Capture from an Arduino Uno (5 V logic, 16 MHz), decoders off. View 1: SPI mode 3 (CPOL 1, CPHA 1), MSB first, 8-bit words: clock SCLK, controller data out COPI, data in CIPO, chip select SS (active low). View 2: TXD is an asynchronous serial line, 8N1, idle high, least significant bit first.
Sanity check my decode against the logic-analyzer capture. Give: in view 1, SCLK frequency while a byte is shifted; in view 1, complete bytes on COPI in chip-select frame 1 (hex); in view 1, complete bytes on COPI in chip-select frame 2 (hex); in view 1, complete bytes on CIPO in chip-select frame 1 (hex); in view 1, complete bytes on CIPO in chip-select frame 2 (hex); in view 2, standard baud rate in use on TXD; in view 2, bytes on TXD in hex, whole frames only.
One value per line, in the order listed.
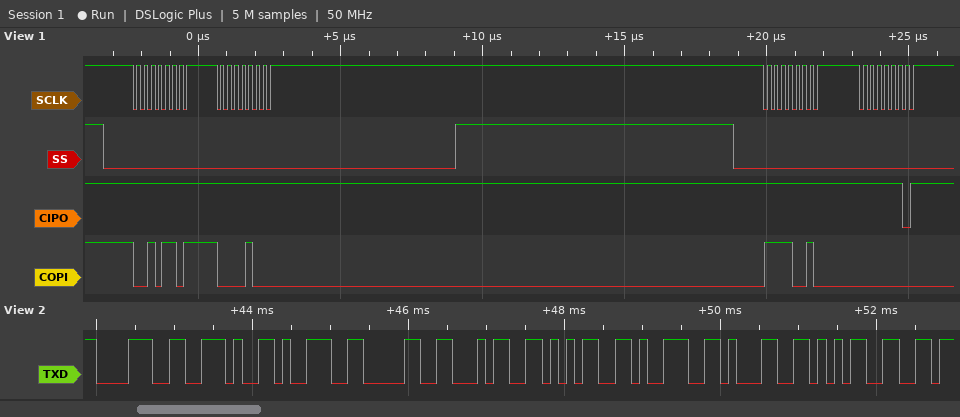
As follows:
4 MHz
2D 08
F2 00
FF FF
FF FD
9600 baud
0x38 0x2E 0x39 0x30 0x34 0x35 0x39 0x31 0x35
